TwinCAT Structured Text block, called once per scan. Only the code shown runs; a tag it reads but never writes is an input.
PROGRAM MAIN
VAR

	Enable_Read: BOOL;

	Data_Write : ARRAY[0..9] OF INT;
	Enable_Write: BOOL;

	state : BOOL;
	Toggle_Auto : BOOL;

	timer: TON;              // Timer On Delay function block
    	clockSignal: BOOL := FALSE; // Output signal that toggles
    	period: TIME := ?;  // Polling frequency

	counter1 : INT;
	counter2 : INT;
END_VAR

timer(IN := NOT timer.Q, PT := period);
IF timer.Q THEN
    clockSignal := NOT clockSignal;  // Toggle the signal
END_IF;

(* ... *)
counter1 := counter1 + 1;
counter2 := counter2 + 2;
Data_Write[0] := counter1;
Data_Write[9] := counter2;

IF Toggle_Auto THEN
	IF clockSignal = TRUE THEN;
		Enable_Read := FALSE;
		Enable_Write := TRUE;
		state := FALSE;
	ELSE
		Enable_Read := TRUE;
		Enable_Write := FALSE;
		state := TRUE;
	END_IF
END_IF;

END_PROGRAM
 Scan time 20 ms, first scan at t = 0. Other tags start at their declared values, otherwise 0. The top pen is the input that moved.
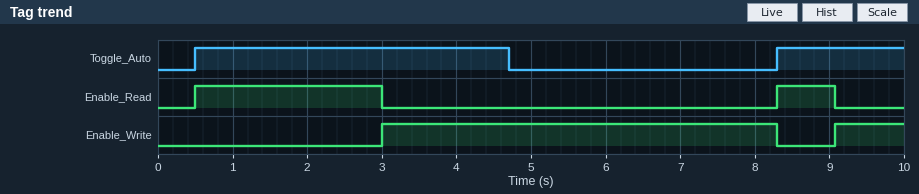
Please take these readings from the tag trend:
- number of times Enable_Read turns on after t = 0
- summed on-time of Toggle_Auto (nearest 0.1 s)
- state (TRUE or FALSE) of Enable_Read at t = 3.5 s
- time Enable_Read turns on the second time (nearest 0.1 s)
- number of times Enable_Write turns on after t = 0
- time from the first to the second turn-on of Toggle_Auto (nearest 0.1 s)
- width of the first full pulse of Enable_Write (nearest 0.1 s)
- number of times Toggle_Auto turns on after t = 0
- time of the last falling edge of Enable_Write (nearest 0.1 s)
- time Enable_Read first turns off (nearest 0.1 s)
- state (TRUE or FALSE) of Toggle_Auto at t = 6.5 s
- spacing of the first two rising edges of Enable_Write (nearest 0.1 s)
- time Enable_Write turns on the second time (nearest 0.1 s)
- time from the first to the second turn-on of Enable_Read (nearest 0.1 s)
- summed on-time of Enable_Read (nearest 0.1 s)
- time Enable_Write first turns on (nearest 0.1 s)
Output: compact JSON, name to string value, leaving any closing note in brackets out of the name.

{"number of times Enable_Read turns on after t = 0": "2", "summed on-time of Toggle_Auto": "5.9 s", "state (TRUE or FALSE) of Enable_Read at t = 3.5 s": "FALSE", "time Enable_Read turns on the second time": "8.3 s", "number of times Enable_Write turns on after t = 0": "2", "time from the first to the second turn-on of Toggle_Auto": "7.8 s", "width of the first full pulse of Enable_Write": "5.3 s", "number of times Toggle_Auto turns on after t = 0": "2", "time of the last falling edge of Enable_Write": "8.3 s", "time Enable_Read first turns off": "3.0 s", "state (TRUE or FALSE) of Toggle_Auto at t = 6.5 s": "FALSE", "spacing of the first two rising edges of Enable_Write": "6.1 s", "time Enable_Write turns on the second time": "9.1 s", "time from the first to the second turn-on of Enable_Read": "7.8 s", "summed on-time of Enable_Read": "3.3 s", "time Enable_Write first turns on": "3.0 s"}
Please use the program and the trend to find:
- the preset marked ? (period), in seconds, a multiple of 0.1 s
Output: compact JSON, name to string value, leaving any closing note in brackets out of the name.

{"the preset marked ? (period), in seconds, a multiple of 0.1 s": "3.0 s"}
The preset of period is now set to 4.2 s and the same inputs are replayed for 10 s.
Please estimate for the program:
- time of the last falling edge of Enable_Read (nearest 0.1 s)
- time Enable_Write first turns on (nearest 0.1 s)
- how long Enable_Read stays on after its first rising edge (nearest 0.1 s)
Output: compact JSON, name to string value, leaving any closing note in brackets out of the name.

{"time of the last falling edge of Enable_Read": "4.2 s", "time Enable_Write first turns on": "4.2 s", "how long Enable_Read stays on after its first rising edge": "3.7 s"}
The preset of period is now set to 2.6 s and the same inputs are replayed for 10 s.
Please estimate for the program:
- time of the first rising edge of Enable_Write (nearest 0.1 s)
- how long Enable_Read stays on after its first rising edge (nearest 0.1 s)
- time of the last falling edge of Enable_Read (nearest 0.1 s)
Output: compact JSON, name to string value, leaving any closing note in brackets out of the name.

{"time of the first rising edge of Enable_Write": "2.6 s", "how long Enable_Read stays on after its first rising edge": "2.1 s", "time of the last falling edge of Enable_Read": "2.6 s"}
